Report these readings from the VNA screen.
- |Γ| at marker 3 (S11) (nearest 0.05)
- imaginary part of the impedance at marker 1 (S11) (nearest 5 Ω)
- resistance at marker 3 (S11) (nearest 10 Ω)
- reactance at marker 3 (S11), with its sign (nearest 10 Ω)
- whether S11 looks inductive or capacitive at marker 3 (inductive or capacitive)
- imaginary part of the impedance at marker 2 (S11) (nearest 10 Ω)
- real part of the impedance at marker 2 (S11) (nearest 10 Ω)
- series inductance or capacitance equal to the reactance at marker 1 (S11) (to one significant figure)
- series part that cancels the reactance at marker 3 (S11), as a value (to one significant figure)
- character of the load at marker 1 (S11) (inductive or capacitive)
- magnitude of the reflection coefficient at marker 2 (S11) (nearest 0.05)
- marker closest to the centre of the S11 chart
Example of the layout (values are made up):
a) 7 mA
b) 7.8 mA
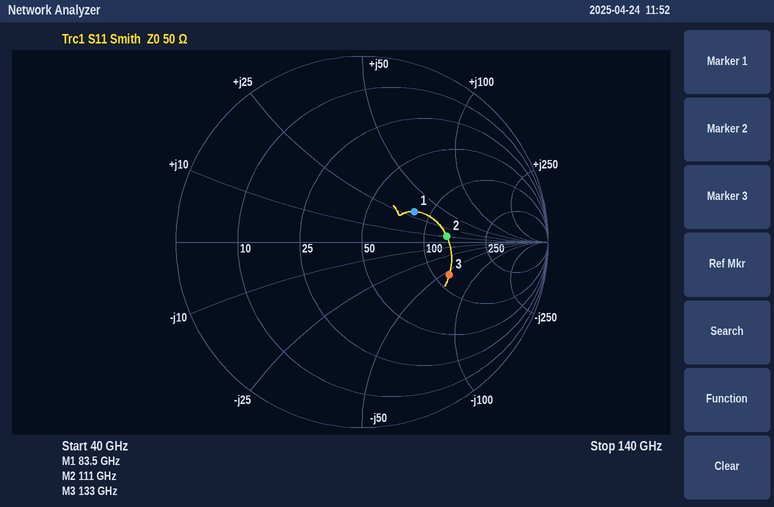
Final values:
a) 0.50
b) +30 Ω
c) 120 Ω
d) -60 Ω
e) capacitive
f) +10 Ω
g) 130 Ω
h) 60 pH
i) 70 pH
j) inductive
k) 0.45
l) marker 1
